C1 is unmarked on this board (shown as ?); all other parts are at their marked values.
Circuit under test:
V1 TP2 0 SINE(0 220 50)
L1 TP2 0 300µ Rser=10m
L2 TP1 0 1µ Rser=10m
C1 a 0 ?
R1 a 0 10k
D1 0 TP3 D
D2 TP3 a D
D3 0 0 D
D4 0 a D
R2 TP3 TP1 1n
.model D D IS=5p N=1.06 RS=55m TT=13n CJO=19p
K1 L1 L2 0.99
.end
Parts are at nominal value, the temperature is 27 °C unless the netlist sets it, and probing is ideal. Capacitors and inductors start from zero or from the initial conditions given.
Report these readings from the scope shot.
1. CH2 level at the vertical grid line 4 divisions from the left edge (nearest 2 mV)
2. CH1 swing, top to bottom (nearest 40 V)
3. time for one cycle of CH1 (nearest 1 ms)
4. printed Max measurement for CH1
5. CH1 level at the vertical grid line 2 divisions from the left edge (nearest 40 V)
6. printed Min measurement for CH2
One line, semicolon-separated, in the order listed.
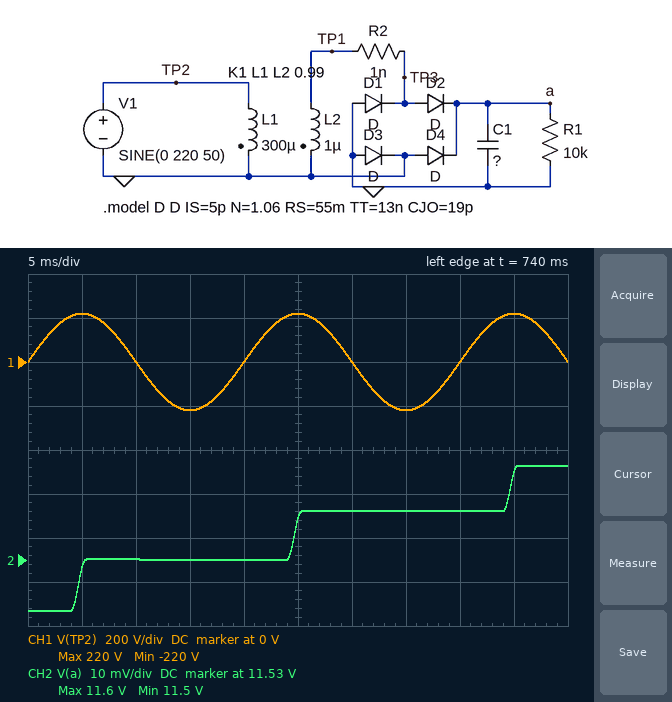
11.530 V; 440 V; 20 ms; 220 V; 0 V; 11.5 V
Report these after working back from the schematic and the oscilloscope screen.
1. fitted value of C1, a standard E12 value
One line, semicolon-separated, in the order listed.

270 mF
